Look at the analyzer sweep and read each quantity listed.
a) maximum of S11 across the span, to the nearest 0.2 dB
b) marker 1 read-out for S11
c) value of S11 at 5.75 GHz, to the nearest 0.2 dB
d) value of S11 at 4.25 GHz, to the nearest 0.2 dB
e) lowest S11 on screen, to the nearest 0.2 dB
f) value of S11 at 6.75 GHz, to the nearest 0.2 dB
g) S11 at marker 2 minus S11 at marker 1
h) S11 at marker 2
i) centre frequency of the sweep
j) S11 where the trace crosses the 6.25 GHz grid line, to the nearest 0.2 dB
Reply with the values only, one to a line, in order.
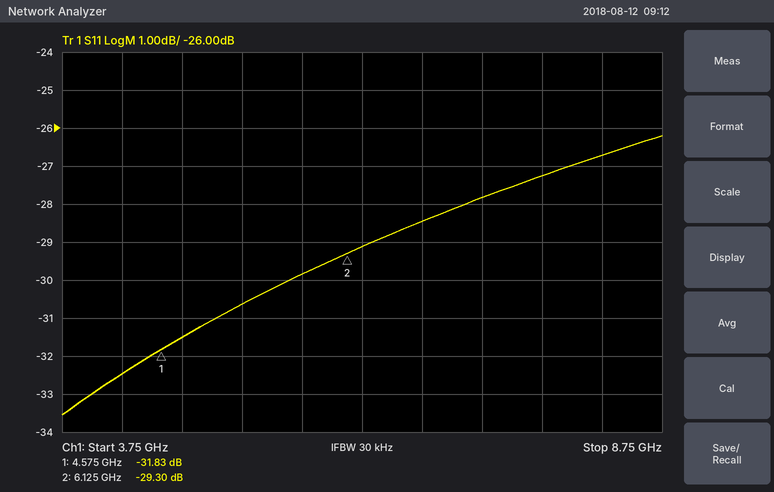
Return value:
-26.2 dB
-31.83 dB
-29.8 dB
-32.4 dB
-33.6 dB
-28.4 dB
2.53 dB
-29.30 dB
6.25 GHz
-29.2 dB
